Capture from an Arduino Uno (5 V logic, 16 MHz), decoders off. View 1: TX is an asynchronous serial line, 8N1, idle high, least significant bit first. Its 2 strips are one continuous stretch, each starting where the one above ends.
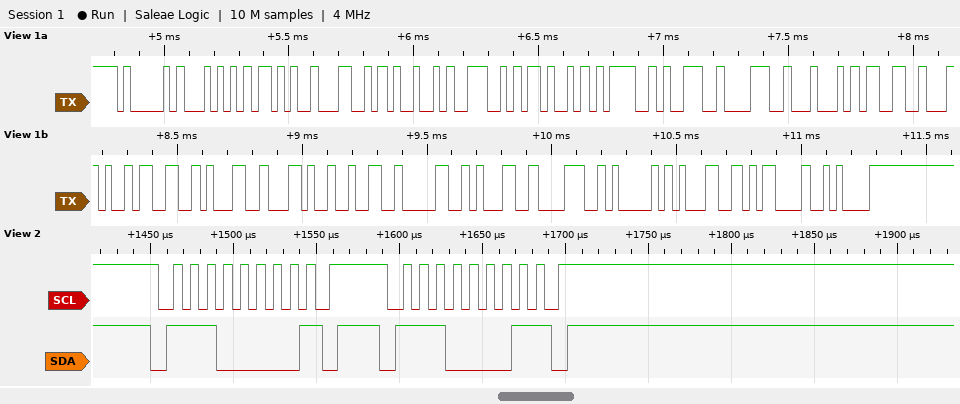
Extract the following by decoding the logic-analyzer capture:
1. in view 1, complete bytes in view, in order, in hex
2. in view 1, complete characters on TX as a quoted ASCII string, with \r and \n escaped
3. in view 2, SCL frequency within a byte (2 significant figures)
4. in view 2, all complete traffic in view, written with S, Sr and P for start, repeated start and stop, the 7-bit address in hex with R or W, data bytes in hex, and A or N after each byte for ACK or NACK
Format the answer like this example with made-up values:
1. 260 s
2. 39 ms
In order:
1. 41 54 2B 4C 49 4E 4B 3D 39 38 44 33 2C 33 31 2C 32 30 31 38 41 31 0D 0A
2. "AT+LINK=98D3,31,2018A1\r\n"
3. 100 kHz
4. S 70W N P S 70R N P
